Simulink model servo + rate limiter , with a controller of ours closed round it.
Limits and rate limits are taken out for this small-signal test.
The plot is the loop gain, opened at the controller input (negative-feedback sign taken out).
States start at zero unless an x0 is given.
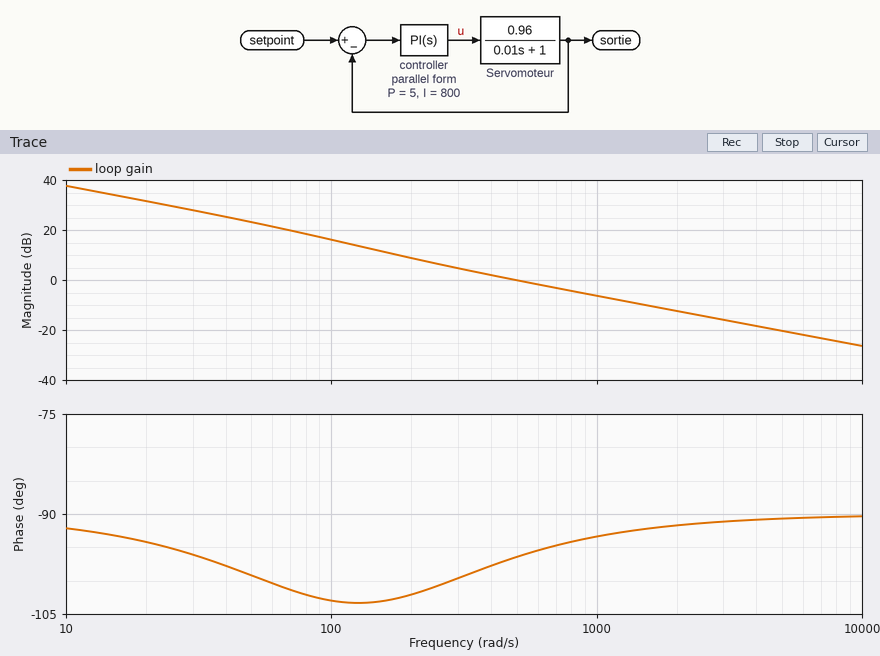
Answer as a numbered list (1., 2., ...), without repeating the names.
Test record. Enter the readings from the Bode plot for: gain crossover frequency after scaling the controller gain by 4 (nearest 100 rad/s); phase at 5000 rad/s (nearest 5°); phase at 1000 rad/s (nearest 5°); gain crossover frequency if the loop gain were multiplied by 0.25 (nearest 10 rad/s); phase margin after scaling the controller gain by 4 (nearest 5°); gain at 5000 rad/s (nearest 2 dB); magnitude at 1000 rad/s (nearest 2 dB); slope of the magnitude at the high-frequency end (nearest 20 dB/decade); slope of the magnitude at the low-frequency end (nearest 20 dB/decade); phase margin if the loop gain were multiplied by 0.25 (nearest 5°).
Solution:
1. 1900 rad/s
2. -90°
3. -95°
4. 150 rad/s
5. 90°
6. -20 dB
7. -6 dB
8. -20 dB/decade
9. -20 dB/decade
10. 75°
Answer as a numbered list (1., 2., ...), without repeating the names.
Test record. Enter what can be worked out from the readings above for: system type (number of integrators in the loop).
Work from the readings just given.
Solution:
1. 1
